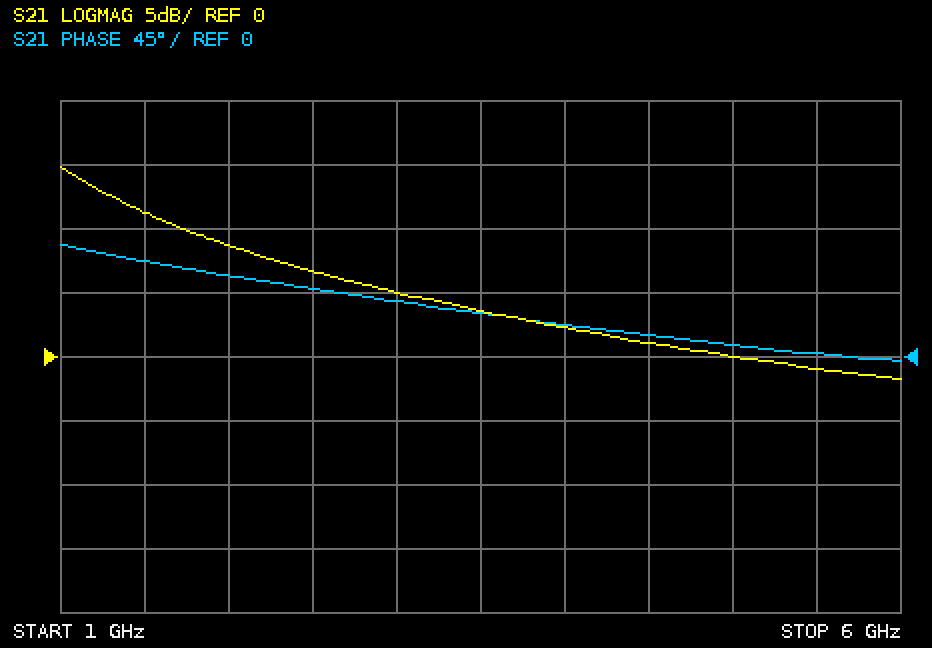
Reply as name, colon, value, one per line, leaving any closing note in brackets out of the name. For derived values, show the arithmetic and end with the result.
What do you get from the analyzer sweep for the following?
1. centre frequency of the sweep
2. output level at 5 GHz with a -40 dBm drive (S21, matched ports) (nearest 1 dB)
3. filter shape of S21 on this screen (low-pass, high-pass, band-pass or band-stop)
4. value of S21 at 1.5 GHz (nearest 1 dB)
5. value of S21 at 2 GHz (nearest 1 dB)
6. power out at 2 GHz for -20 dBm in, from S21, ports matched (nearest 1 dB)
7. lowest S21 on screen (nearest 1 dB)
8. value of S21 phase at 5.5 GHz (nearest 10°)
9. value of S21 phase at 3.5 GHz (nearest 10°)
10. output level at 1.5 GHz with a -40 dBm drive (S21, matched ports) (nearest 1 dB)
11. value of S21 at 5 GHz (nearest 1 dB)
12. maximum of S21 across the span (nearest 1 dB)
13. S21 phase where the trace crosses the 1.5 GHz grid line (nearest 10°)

centre frequency of the sweep: 3.5 GHz
output level at 5 GHz with a -40 dBm drive (S21, matched ports): -40 dBm + (0 dB) = -40 dBm
filter shape of S21 on this screen: low-pass
value of S21 at 1.5 GHz: 11 dB
value of S21 at 2 GHz: 9 dB
power out at 2 GHz for -20 dBm in, from S21, ports matched: -20 dBm + (9 dB) = -11 dBm
lowest S21 on screen: -2 dB
value of S21 phase at 5.5 GHz: 0°
value of S21 phase at 3.5 GHz: 30°
output level at 1.5 GHz with a -40 dBm drive (S21, matched ports): -40 dBm + (11 dB) = -29 dBm
value of S21 at 5 GHz: 0 dB
maximum of S21 across the span: 15 dB
S21 phase where the trace crosses the 1.5 GHz grid line: 70°
